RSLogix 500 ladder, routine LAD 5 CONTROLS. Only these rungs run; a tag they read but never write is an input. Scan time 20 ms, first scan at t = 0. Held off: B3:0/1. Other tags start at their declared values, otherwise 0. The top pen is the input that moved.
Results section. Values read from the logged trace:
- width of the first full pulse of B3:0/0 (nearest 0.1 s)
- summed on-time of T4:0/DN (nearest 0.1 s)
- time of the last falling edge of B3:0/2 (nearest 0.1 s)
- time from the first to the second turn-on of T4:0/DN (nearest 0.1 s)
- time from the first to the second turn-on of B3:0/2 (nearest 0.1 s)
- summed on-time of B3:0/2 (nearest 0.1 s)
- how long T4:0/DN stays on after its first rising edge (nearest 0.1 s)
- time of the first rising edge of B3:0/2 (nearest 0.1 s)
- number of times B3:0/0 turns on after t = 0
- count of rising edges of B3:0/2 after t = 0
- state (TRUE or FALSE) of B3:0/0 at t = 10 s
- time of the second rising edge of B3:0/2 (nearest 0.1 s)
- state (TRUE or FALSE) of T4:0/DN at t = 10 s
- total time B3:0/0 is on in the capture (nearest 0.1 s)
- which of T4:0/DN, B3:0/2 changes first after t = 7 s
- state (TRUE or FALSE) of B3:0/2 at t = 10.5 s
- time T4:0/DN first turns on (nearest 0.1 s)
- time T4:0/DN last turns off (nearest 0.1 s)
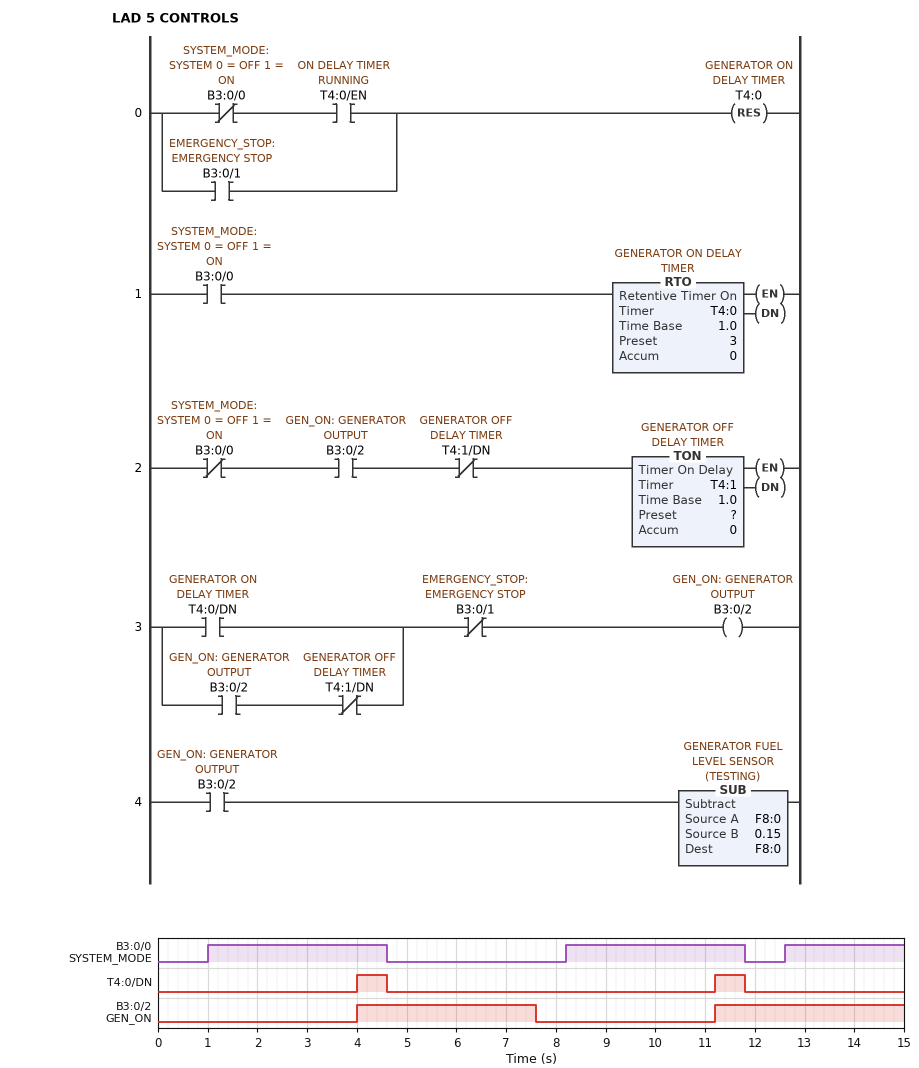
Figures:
3.6 s
1.2 s
7.6 s
7.2 s
7.2 s
7.4 s
0.6 s
4.0 s
3
2
TRUE
11.2 s
FALSE
9.6 s
B3:0/2
FALSE
4.0 s
11.8 s
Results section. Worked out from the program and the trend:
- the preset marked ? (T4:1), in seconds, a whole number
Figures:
3 s
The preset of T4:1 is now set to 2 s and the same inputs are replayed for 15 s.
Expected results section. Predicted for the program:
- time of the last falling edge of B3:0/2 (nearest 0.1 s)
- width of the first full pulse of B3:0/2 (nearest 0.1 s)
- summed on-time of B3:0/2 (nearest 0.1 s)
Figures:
6.6 s
2.6 s
6.4 s
